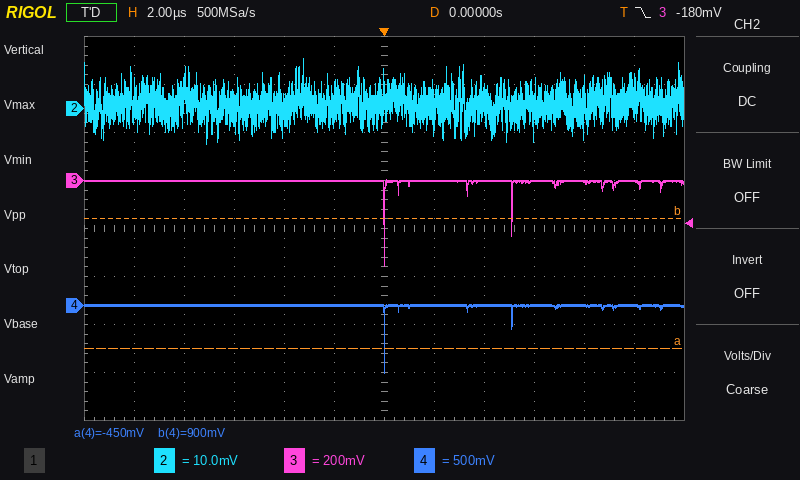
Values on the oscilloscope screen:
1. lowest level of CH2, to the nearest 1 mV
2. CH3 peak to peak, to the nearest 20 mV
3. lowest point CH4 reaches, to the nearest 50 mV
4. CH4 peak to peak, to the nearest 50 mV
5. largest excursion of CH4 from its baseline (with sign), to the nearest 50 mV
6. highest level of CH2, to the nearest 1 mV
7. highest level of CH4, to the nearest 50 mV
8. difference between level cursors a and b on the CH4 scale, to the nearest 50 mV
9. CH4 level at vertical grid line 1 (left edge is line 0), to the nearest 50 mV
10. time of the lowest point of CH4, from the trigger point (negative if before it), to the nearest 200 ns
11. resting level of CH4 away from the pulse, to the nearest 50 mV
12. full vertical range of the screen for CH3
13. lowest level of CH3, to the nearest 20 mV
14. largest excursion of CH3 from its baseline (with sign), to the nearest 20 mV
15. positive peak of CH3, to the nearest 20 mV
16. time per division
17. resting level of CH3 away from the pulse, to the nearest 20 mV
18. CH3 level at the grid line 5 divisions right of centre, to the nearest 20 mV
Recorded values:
-7 mV
360 mV
-700 mV
700 mV
-700 mV
10 mV
0 mV
1.35 V
0 mV
0.0 µs
0 mV
1.6 V
-360 mV
-360 mV
0 mV
2 µs
0 mV
0 mV
